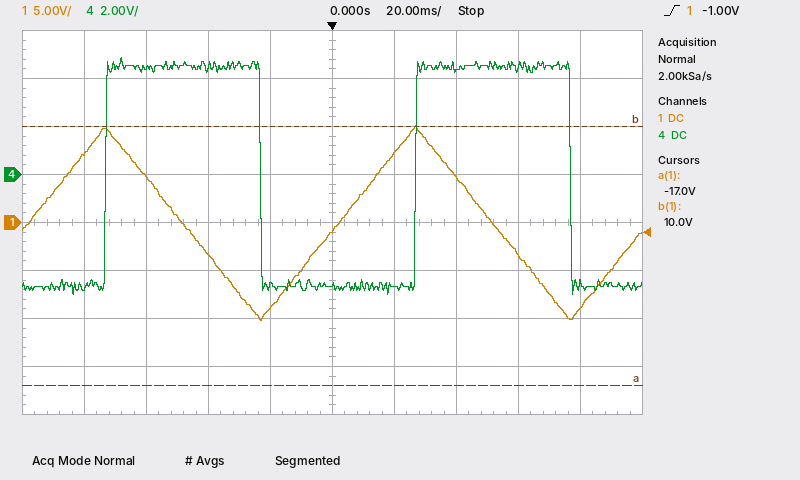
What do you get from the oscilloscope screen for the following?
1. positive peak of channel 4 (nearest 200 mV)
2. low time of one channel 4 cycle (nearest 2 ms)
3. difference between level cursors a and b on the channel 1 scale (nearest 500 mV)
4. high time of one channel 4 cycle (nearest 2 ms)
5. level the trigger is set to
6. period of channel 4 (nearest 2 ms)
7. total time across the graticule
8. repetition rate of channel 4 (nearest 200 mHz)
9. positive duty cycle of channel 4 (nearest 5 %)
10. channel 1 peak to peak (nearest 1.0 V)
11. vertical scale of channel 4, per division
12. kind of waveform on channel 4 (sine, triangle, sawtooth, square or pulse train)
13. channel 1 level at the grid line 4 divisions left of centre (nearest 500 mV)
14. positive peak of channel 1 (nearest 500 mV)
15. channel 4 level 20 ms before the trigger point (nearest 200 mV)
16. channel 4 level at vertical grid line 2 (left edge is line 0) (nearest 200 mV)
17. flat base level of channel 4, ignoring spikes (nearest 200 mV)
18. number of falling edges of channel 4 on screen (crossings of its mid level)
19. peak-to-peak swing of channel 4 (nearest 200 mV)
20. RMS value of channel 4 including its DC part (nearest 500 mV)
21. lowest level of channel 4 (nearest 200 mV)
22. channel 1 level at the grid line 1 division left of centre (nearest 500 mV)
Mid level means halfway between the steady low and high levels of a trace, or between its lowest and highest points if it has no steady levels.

4.8 V
50 ms
27.0 V
50 ms
-1.00 V
100 ms
200 ms
10.0 Hz
50 %
20.0 V
2 V
square
7.0 V
10.0 V
-4.6 V
4.4 V
-4.6 V
2
9.8 V
4.5 V
-5.0 V
-9.0 V
